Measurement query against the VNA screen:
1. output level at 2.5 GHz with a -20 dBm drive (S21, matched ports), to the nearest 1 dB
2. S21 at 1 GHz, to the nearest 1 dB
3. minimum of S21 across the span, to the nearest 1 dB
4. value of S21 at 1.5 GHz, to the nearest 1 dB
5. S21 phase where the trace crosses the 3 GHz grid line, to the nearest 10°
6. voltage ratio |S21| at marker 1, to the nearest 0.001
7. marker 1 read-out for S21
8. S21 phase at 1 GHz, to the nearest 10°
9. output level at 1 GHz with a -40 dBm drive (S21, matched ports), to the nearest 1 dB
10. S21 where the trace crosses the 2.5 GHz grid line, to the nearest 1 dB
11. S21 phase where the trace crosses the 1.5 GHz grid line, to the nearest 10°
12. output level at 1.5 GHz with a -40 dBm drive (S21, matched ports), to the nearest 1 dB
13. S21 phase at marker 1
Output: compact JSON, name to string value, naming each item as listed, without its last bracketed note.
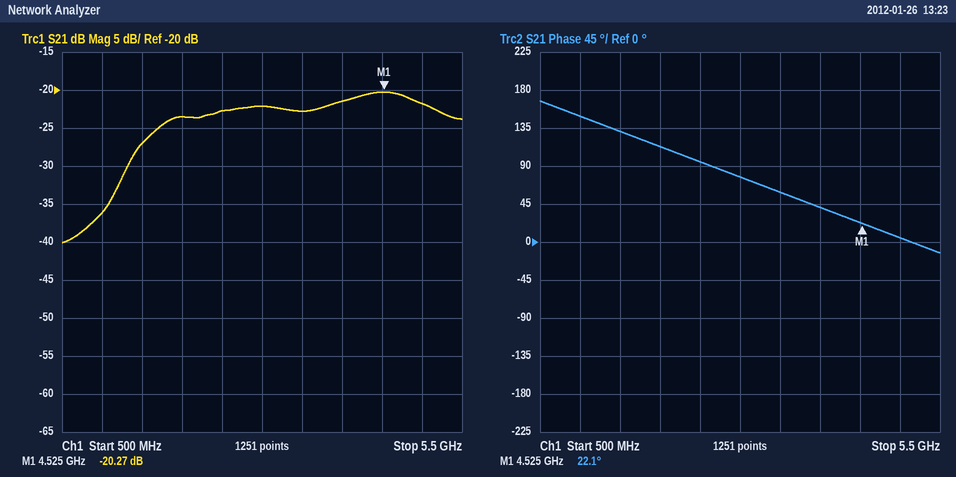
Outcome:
{"output level at 2.5 GHz with a -20 dBm drive (S21, matched ports), to the nearest 1 dB": "-43 dBm", "S21 at 1 GHz, to the nearest 1 dB": "-36 dB", "minimum of S21 across the span, to the nearest 1 dB": "-40 dB", "value of S21 at 1.5 GHz, to the nearest 1 dB": "-27 dB", "S21 phase where the trace crosses the 3 GHz grid line, to the nearest 10°": "80°", "voltage ratio |S21| at marker 1, to the nearest 0.001": "0.097", "marker 1 read-out for S21": "-20.27 dB", "S21 phase at 1 GHz, to the nearest 10°": "150°", "output level at 1 GHz with a -40 dBm drive (S21, matched ports), to the nearest 1 dB": "-76 dBm", "S21 where the trace crosses the 2.5 GHz grid line, to the nearest 1 dB": "-23 dB", "S21 phase where the trace crosses the 1.5 GHz grid line, to the nearest 10°": "130°", "output level at 1.5 GHz with a -40 dBm drive (S21, matched ports), to the nearest 1 dB": "-67 dBm", "S21 phase at marker 1": "22.1°"}
